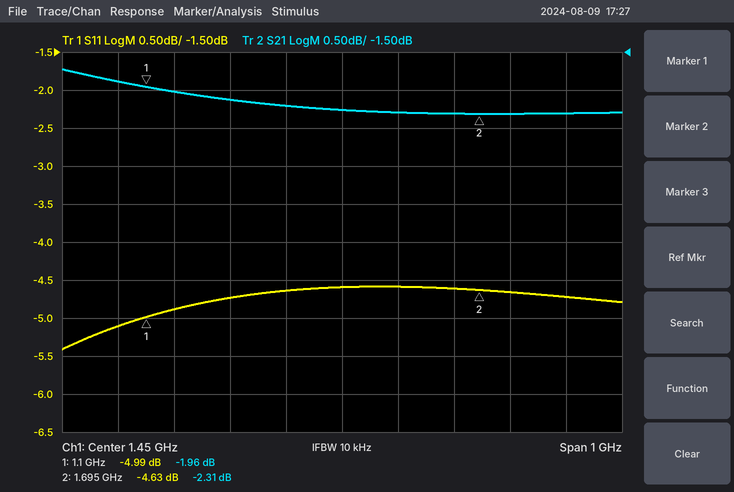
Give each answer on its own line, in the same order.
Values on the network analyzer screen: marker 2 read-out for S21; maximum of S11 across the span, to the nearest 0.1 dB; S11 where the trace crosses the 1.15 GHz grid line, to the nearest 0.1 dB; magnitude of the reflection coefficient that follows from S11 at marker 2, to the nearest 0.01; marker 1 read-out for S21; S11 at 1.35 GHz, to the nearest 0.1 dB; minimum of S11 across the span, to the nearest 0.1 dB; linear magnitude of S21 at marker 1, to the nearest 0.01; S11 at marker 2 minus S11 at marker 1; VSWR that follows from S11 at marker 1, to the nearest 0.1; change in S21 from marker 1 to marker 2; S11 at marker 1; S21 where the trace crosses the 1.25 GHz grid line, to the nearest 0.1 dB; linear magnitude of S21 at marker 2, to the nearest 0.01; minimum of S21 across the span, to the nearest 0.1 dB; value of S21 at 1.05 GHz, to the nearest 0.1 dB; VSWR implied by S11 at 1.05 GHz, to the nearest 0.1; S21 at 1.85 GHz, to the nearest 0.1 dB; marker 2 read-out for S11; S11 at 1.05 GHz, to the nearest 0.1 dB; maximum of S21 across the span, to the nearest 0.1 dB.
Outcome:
-2.31 dB
-4.6 dB
-4.9 dB
0.59
-1.96 dB
-4.6 dB
-5.4 dB
0.80
0.36 dB
3.6
-0.35 dB
-4.99 dB
-2.1 dB
0.77
-2.3 dB
-1.9 dB
3.5
-2.3 dB
-4.63 dB
-5.1 dB
-1.7 dB
